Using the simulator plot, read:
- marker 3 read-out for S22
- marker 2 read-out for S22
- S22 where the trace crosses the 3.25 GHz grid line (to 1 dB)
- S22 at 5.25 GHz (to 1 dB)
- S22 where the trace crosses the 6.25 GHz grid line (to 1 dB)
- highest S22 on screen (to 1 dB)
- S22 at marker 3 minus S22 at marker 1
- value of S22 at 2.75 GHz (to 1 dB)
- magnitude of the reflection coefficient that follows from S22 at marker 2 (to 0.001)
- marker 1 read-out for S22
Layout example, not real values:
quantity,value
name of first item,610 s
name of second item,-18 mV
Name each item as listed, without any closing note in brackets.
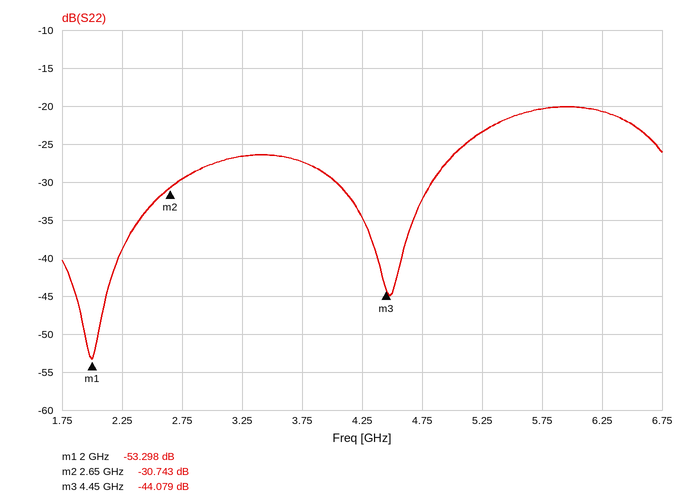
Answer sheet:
quantity,value
marker 3 read-out for S22,-44.079 dB
marker 2 read-out for S22,-30.743 dB
S22 where the trace crosses the 3.25 GHz grid line,-27 dB
S22 at 5.25 GHz,-23 dB
S22 where the trace crosses the 6.25 GHz grid line,-21 dB
highest S22 on screen,-20 dB
S22 at marker 3 minus S22 at marker 1,9.219 dB
value of S22 at 2.75 GHz,-30 dB
magnitude of the reflection coefficient that follows from S22 at marker 2,0.029
marker 1 read-out for S22,-53.298 dB
